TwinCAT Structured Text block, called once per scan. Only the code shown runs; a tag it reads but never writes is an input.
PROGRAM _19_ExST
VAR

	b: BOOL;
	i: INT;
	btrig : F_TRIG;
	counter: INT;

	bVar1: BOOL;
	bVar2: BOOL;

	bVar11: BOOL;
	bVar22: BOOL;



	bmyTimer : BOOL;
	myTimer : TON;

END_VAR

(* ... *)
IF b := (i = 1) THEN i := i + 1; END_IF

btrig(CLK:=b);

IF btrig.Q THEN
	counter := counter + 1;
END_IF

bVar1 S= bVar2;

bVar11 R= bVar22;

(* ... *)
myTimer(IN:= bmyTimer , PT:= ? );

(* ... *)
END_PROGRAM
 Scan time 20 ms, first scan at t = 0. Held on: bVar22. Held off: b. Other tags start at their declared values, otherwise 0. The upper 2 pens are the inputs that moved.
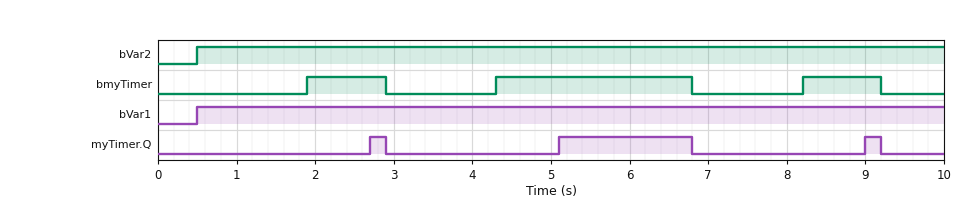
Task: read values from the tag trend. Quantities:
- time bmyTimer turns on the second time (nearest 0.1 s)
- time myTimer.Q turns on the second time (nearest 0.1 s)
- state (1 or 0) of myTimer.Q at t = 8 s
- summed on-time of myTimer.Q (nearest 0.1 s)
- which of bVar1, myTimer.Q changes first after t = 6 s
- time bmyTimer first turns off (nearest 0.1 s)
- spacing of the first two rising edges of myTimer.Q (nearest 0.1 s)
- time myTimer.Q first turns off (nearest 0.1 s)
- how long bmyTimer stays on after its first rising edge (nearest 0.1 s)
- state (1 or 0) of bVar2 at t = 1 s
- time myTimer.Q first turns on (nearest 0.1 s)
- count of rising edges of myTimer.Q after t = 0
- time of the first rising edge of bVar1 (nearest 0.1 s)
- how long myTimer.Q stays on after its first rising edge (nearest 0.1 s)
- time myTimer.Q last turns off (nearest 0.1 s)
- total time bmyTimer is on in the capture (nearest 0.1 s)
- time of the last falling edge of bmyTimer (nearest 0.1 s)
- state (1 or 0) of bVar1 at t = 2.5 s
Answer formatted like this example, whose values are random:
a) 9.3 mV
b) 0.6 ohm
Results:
a) 4.3 s
b) 5.1 s
c) 0
d) 2.1 s
e) myTimer.Q
f) 2.9 s
g) 2.4 s
h) 2.9 s
i) 1.0 s
j) 1
k) 2.7 s
l) 3
m) 0.5 s
n) 0.2 s
o) 9.2 s
p) 4.5 s
q) 9.2 s
r) 1
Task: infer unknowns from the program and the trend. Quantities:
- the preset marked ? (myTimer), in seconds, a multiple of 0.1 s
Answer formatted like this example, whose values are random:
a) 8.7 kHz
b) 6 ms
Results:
a) 0.8 s
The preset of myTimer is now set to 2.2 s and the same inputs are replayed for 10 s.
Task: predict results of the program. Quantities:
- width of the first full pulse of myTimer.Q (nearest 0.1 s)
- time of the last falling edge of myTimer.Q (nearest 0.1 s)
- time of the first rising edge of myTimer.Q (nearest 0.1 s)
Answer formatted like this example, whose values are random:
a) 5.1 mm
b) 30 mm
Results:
a) 0.3 s
b) 6.8 s
c) 6.5 s
